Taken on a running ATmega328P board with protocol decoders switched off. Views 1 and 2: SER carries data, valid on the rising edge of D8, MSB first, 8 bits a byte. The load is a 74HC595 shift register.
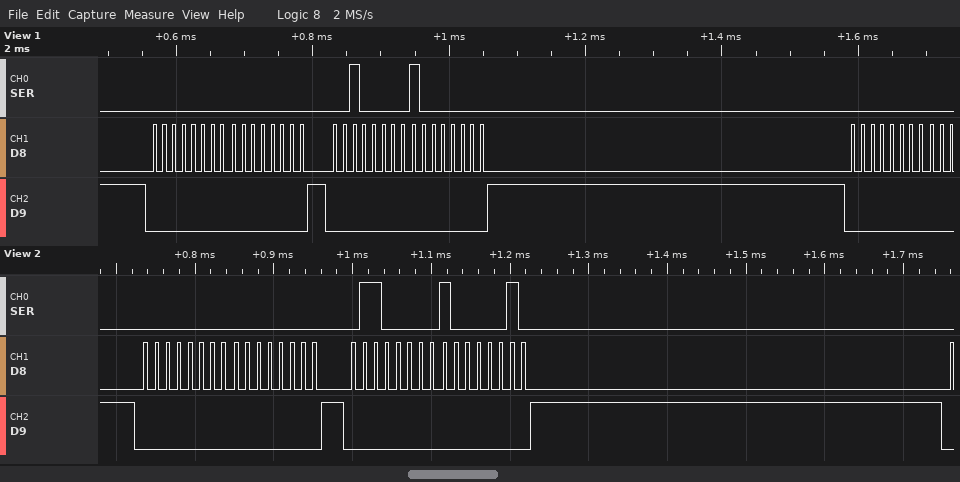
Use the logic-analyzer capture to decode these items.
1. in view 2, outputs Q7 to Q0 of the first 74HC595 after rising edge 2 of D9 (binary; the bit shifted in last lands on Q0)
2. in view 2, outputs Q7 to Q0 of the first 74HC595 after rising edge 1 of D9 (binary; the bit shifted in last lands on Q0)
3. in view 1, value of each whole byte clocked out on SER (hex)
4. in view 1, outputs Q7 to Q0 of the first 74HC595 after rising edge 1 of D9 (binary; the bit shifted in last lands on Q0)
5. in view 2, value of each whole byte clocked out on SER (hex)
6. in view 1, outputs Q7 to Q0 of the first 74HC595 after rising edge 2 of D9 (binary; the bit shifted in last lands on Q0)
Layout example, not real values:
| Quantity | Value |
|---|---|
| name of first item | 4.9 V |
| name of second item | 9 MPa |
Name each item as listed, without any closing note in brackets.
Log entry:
| Quantity | Value |
|---|---|
| in view 2, outputs Q7 to Q0 of the first 74HC595 after rising edge 2 of D9 | 10000010 |
| in view 2, outputs Q7 to Q0 of the first 74HC595 after rising edge 1 of D9 | 00000000 |
| in view 1, value of each whole byte clocked out on SER | 00 00 20 80 00 |
| in view 1, outputs Q7 to Q0 of the first 74HC595 after rising edge 1 of D9 | 00000000 |
| in view 2, value of each whole byte clocked out on SER | 00 00 60 82 |
| in view 1, outputs Q7 to Q0 of the first 74HC595 after rising edge 2 of D9 | 10000000 |
